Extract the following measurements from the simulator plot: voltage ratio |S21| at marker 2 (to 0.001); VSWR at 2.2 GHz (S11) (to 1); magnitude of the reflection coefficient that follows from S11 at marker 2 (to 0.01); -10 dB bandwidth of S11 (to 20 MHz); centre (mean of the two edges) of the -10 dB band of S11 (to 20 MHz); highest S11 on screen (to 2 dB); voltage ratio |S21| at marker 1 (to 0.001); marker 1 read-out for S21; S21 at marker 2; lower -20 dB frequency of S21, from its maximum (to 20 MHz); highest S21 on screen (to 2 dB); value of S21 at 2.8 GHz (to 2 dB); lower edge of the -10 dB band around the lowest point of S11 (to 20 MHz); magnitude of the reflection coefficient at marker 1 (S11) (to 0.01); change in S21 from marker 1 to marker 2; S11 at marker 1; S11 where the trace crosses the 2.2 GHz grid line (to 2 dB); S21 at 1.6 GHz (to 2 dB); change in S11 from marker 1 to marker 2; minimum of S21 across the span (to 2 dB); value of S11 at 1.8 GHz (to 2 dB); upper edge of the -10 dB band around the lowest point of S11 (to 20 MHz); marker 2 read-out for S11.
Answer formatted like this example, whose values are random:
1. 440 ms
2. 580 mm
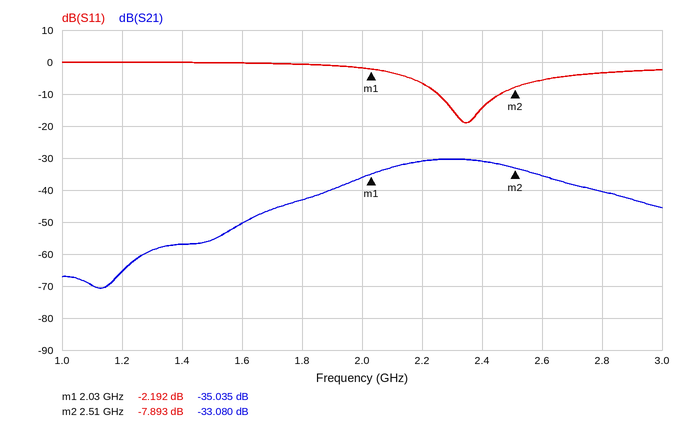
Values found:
1. 0.022
2. 3
3. 0.40
4. 200 MHz
5. 2.36 GHz
6. 0 dB
7. 0.018
8. -35.035 dB
9. -33.080 dB
10. 1.60 GHz
11. -30 dB
12. -40 dB
13. 2.26 GHz
14. 0.78
15. 1.955 dB
16. -2.192 dB
17. -6 dB
18. -50 dB
19. -5.701 dB
20. -70 dB
21. 0 dB
22. 2.46 GHz
23. -7.893 dB
